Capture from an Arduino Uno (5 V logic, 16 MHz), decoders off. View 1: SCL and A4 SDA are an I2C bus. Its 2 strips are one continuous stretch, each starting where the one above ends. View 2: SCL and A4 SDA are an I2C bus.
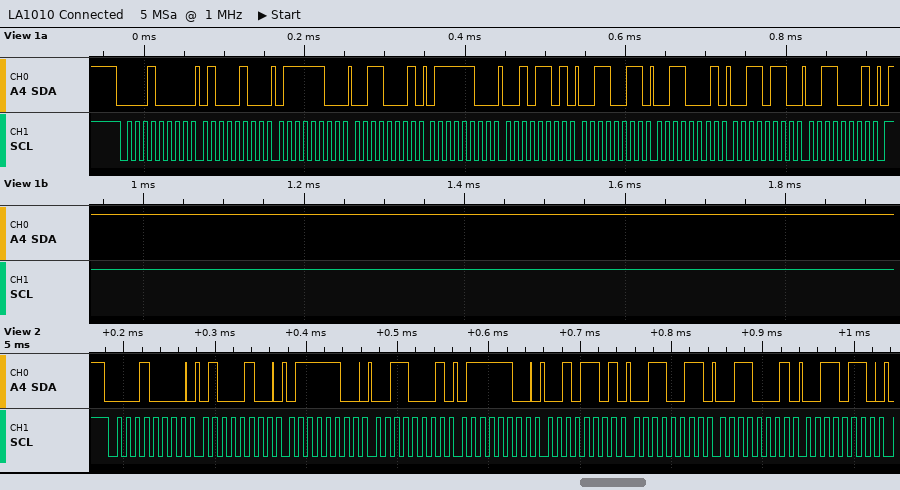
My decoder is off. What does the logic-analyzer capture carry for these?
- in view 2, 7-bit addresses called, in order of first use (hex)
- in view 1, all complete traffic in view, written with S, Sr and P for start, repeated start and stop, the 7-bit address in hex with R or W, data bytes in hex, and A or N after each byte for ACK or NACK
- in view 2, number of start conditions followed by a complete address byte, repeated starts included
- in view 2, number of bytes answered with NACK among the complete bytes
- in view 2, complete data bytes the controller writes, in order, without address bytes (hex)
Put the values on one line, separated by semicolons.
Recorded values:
0x08; S 08W A 44 A 7C A 31 A 7C A 2D A 33 A 31 A 36 A 31 A P; 1; 0; 44 7C 31 7C 2D 33 31 36
